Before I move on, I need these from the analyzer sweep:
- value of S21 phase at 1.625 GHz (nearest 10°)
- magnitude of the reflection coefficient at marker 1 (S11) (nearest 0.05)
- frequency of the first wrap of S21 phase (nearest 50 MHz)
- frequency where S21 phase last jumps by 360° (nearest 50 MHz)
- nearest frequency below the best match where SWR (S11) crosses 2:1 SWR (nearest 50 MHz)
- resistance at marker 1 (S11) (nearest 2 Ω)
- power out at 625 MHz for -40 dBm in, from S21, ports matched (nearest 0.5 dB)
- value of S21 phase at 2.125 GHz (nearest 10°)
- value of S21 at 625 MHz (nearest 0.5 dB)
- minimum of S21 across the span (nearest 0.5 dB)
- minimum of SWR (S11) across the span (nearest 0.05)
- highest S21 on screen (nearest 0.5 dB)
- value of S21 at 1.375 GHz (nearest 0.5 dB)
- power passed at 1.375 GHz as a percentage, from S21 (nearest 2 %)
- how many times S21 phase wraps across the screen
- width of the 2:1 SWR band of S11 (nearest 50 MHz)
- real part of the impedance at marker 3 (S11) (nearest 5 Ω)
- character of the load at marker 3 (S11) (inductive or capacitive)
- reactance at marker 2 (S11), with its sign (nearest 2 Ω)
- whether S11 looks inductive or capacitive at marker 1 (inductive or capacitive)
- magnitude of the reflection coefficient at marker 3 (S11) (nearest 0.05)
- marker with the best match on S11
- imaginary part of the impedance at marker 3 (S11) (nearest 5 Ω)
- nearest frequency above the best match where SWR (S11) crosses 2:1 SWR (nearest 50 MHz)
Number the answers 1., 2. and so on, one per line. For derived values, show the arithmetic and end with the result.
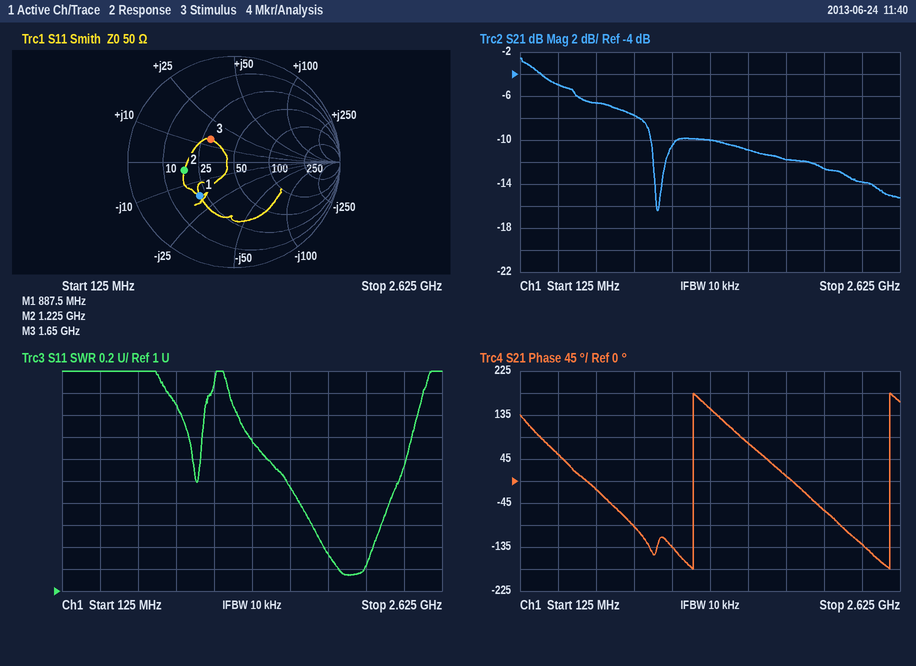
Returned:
1. 80°
2. 0.45
3. 1.25 GHz
4. 2.55 GHz
5. 1.60 GHz
6. 22 Ω
7. -40 dBm + (-6.5 dB) = -46.5 dBm
8. -60°
9. -6.5 dB
10. -16.5 dB
11. 1.15
12. -2.5 dB
13. -10.0 dB
14. 10^(-10/10) ≈ 10 %
15. 2
16. 2.35 GHz − 1.60 GHz = 750 MHz
17. 30 Ω
18. inductive
19. -4 Ω
20. capacitive
21. 0.30
22. marker 3
23. +15 Ω
24. 2.35 GHz
